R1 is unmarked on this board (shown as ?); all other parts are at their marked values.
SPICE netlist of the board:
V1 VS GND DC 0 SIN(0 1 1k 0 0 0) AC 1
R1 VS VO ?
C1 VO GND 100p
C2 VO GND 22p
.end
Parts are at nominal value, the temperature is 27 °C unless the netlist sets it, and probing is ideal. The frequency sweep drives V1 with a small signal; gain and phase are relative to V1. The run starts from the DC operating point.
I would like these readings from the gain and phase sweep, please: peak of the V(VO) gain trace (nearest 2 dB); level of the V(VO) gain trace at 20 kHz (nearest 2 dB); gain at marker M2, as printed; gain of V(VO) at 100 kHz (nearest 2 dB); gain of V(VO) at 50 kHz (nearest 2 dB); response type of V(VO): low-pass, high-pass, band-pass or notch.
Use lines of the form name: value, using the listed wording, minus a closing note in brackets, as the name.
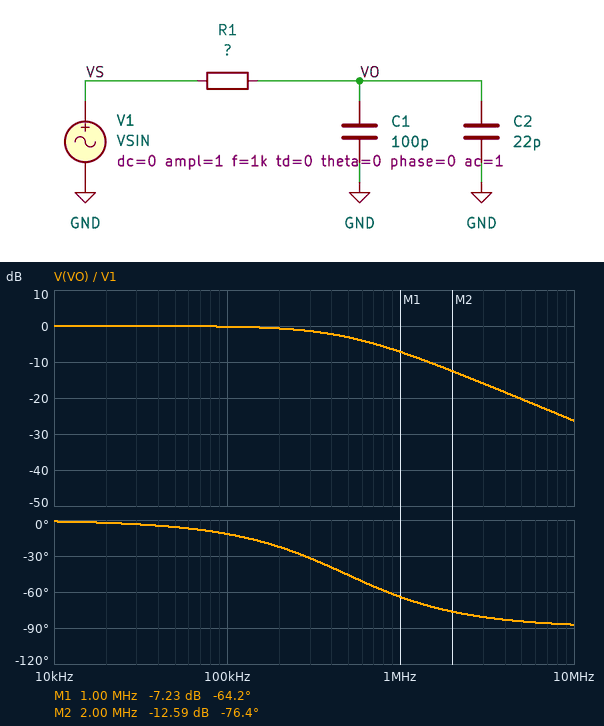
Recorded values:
peak of the V(VO) gain trace: 0 dB
level of the V(VO) gain trace at 20 kHz: 0 dB
gain at marker M2, as printed: -12.59 dB
gain of V(VO) at 100 kHz: 0 dB
gain of V(VO) at 50 kHz: 0 dB
response type of V(VO): low-pass, high-pass, band-pass or notch: low-pass
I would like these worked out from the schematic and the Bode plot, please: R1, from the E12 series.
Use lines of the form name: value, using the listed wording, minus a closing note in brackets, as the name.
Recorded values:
R1, from the E12 series: 2.7 kΩ
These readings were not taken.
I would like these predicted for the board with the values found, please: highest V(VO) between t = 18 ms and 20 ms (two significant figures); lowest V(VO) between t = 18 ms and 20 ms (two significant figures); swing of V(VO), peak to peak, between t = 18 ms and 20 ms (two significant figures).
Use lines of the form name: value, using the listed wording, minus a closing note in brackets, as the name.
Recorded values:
highest V(VO) between t = 18 ms and 20 ms: 1.0 V
lowest V(VO) between t = 18 ms and 20 ms: -1.0 V
swing of V(VO), peak to peak, between t = 18 ms and 20 ms: 2.0 V
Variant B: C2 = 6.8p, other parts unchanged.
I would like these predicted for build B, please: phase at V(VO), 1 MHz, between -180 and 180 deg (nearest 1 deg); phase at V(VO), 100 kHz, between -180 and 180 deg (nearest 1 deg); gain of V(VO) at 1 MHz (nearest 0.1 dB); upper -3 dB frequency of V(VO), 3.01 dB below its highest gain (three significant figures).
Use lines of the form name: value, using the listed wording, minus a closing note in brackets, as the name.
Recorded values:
phase at V(VO), 1 MHz, between -180 and 180 deg: -61 deg
phase at V(VO), 100 kHz, between -180 and 180 deg: -10 deg
gain of V(VO) at 1 MHz: -6.3 dB
upper -3 dB frequency of V(VO), 3.01 dB below its highest gain: 552 kHz
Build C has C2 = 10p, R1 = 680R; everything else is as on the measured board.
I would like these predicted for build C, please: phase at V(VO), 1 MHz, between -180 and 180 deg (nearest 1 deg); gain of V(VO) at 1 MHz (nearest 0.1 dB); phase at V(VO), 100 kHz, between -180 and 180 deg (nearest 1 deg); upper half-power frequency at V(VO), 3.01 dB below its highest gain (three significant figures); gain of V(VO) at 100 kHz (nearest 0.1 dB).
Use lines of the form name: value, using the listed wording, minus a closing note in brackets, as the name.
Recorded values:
phase at V(VO), 1 MHz, between -180 and 180 deg: -25 deg
gain of V(VO) at 1 MHz: -0.9 dB
phase at V(VO), 100 kHz, between -180 and 180 deg: -3 deg
upper half-power frequency at V(VO), 3.01 dB below its highest gain: 2.13 MHz
gain of V(VO) at 100 kHz: 0 dB
